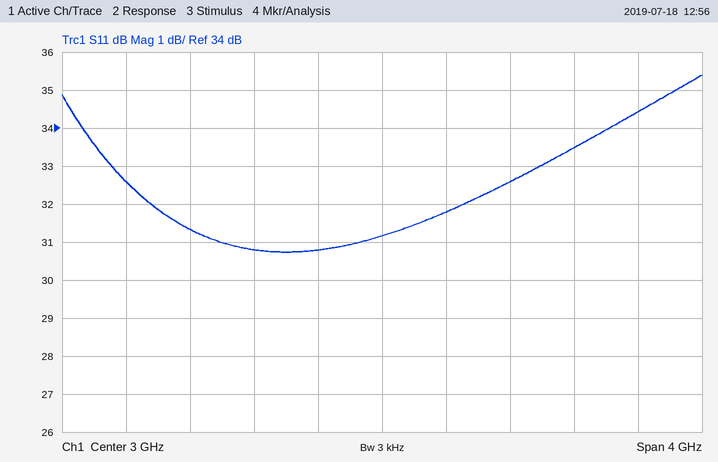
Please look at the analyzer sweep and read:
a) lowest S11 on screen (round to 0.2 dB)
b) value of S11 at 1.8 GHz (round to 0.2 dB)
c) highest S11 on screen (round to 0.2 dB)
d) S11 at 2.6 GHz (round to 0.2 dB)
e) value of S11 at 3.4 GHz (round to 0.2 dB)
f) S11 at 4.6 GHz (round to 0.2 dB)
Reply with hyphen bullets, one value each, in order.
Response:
- 30.8 dB
- 31.4 dB
- 35.4 dB
- 30.8 dB
- 31.8 dB
- 34.4 dB
